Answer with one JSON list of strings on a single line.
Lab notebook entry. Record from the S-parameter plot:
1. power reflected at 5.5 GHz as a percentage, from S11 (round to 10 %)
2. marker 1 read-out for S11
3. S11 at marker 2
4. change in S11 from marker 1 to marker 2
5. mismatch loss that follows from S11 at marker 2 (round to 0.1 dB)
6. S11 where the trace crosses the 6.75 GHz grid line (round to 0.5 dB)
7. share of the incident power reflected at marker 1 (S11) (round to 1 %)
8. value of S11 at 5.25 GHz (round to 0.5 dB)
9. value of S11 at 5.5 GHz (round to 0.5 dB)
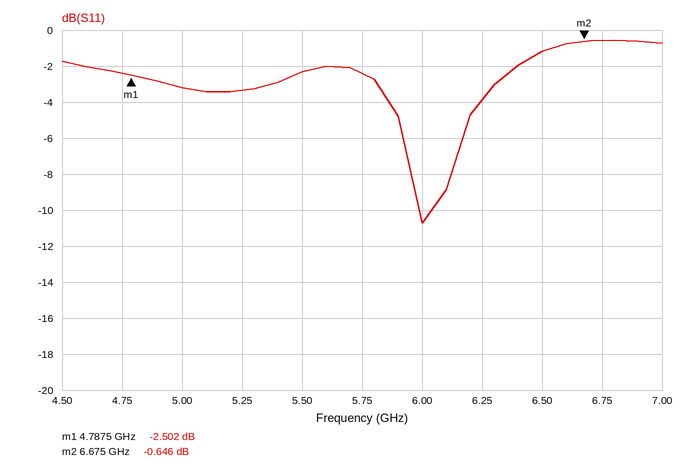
["60 %", "-2.502 dB", "-0.646 dB", "1.856 dB", "8.6 dB", "-0.5 dB", "56 %", "-3.5 dB", "-2.5 dB"]
